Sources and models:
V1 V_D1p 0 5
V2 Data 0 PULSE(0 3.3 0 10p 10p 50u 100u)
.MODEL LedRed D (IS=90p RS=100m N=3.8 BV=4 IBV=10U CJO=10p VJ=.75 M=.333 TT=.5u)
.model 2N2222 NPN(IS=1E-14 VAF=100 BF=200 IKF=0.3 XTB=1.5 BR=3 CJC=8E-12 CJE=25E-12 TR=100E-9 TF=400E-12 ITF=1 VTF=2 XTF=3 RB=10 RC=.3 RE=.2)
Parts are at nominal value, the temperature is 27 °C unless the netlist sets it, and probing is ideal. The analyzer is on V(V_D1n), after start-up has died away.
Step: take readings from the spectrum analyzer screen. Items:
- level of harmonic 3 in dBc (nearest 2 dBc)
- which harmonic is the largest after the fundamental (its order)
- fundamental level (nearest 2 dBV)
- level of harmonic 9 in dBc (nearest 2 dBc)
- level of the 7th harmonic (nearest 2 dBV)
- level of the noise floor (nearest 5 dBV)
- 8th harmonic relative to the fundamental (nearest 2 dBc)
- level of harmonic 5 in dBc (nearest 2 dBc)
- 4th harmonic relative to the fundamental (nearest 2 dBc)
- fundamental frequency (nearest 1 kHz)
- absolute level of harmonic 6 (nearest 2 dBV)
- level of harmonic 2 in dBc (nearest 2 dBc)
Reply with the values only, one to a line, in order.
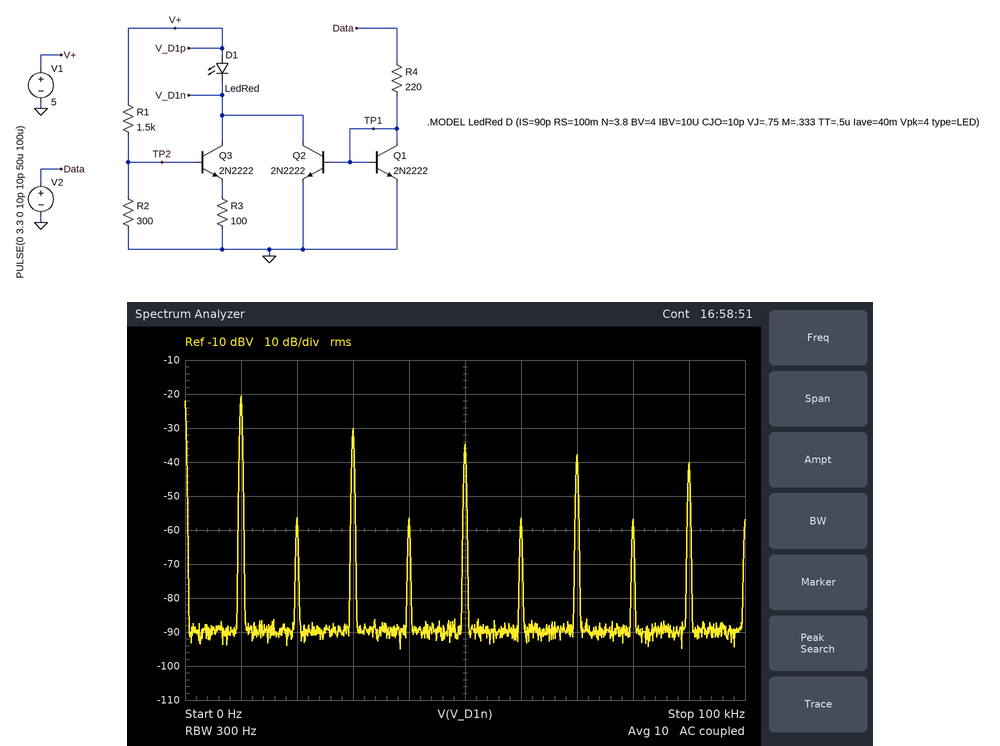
-10 dBc
3
-20 dBV
-20 dBc
-38 dBV
-90 dBV
-36 dBc
-14 dBc
-36 dBc
10 kHz
-56 dBV
-36 dBc
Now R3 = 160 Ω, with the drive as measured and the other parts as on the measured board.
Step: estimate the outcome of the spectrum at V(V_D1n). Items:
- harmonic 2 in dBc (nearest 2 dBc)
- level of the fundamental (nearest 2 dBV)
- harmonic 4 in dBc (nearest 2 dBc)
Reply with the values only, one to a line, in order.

-34 dBc
-20 dBV
-34 dBc
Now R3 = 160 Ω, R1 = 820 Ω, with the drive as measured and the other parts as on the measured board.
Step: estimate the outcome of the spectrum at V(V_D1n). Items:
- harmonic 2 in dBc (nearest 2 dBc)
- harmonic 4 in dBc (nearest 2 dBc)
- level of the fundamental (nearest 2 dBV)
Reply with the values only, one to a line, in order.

-40 dBc
-40 dBc
-24 dBV
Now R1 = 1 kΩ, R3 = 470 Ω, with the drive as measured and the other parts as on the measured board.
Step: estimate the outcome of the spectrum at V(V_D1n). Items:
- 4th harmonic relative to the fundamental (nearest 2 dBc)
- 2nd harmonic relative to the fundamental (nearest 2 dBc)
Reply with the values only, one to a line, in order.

-34 dBc
-34 dBc
